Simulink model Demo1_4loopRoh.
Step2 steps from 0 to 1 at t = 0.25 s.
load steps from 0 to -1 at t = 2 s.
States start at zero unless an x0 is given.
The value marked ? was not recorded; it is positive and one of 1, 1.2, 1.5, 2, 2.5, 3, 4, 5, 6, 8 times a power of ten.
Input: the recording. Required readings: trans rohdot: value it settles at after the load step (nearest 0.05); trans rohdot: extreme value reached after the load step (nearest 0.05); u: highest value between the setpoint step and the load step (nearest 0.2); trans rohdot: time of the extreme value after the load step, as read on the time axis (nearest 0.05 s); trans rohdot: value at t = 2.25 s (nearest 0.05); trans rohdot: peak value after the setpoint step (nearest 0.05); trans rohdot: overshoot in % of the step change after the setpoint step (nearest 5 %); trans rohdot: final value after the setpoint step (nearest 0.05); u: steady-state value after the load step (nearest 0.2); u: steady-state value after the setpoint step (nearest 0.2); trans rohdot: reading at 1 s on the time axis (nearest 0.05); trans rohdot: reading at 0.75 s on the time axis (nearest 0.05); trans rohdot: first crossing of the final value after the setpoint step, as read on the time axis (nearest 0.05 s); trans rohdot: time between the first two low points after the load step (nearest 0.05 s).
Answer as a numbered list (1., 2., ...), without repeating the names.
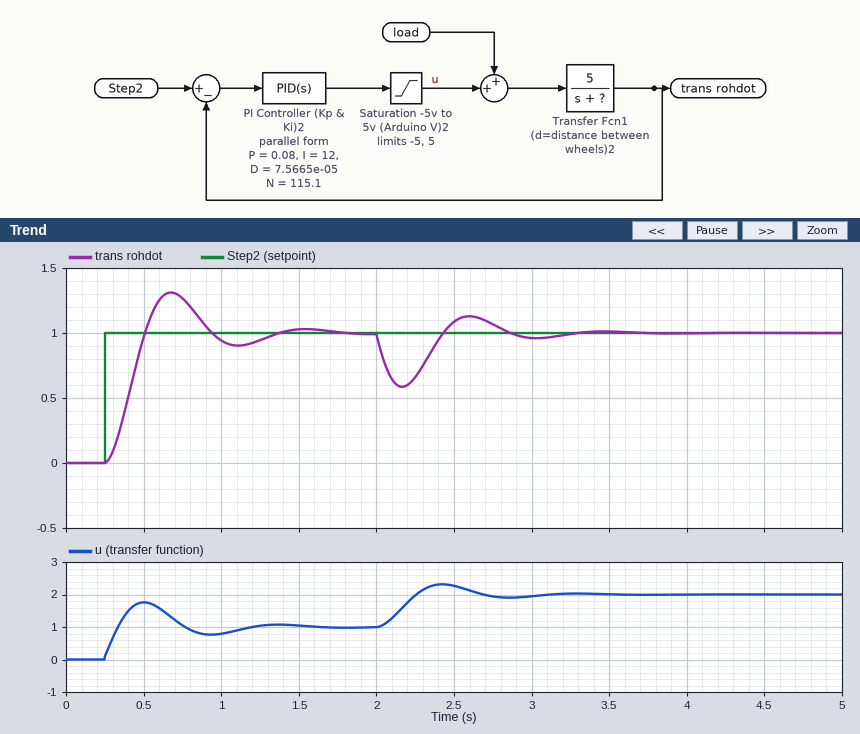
1. 1.00
2. 0.60
3. 1.8
4. 2.15 s
5. 0.65
6. 1.30
7. 30 %
8. 1.00
9. 2.0
10. 1.0
11. 0.95
12. 1.25
13. 0.50 s
14. 0.85 s
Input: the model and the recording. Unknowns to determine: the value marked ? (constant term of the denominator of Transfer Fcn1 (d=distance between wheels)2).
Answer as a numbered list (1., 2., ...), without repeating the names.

1. 5
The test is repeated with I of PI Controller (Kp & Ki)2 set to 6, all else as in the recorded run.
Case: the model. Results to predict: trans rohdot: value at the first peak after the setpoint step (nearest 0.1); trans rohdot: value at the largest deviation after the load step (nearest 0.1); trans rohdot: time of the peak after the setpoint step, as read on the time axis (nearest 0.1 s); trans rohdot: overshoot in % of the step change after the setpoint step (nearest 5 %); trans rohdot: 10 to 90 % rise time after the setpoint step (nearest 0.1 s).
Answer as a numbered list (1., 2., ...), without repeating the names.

1. 1.2
2. 0.5
3. 0.9 s
4. 15 %
5. 0.3 s
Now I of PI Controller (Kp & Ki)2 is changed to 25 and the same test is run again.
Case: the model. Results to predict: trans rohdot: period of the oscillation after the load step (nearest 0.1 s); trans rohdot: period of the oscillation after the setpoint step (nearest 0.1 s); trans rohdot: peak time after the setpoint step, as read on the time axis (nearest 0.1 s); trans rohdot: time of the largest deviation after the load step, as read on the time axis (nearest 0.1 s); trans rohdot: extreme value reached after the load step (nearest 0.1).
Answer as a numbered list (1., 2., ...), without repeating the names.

1. 0.6 s
2. 0.6 s
3. 0.5 s
4. 2.1 s
5. 0.7
